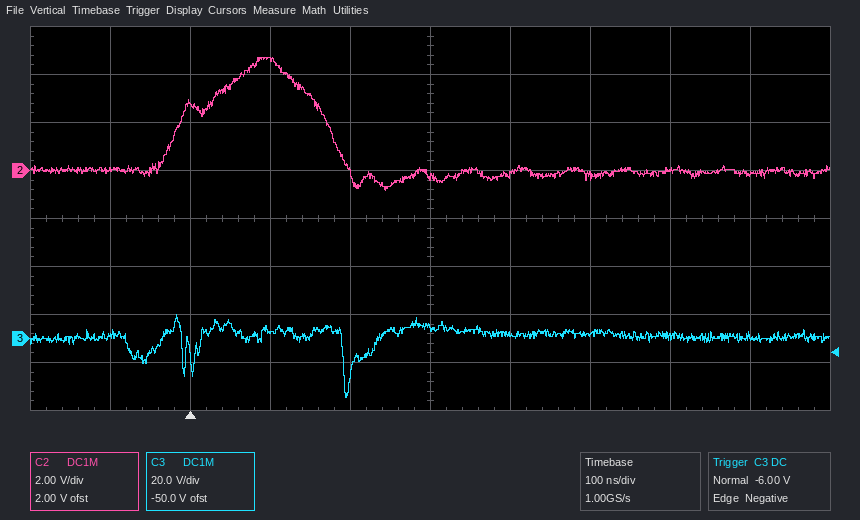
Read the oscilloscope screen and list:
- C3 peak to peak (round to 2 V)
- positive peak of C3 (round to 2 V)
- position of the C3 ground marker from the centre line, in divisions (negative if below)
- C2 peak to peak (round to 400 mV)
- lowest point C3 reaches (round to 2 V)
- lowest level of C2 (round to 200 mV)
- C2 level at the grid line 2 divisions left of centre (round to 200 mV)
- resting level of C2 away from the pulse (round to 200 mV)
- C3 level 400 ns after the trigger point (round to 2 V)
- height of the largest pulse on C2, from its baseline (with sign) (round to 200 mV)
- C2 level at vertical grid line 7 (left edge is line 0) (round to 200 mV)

34 V
10 V
-2.5 div
5.6 V
-24 V
-800 mV
4.6 V
0.0 V
2 V
+4.8 V
-200 mV
